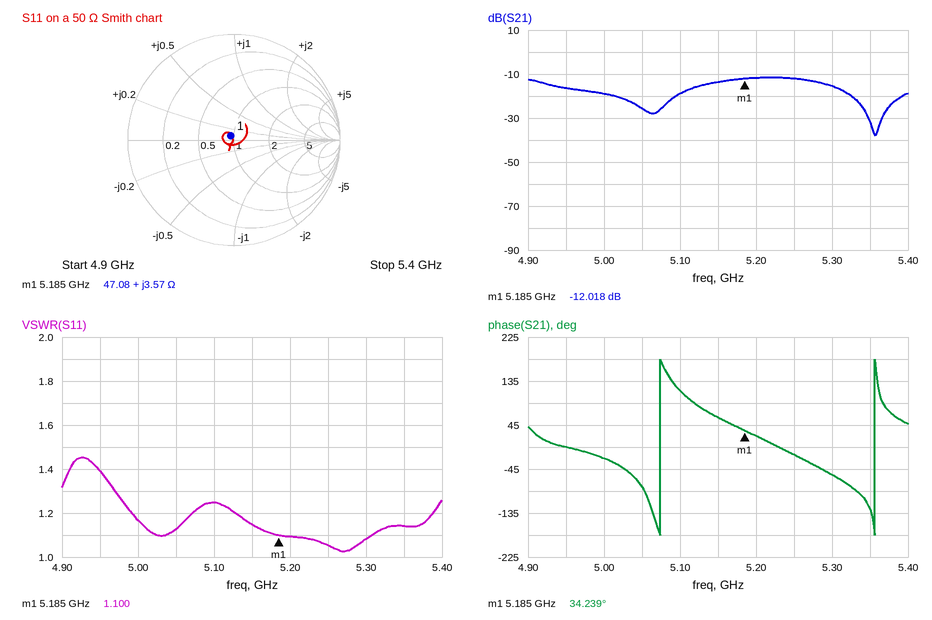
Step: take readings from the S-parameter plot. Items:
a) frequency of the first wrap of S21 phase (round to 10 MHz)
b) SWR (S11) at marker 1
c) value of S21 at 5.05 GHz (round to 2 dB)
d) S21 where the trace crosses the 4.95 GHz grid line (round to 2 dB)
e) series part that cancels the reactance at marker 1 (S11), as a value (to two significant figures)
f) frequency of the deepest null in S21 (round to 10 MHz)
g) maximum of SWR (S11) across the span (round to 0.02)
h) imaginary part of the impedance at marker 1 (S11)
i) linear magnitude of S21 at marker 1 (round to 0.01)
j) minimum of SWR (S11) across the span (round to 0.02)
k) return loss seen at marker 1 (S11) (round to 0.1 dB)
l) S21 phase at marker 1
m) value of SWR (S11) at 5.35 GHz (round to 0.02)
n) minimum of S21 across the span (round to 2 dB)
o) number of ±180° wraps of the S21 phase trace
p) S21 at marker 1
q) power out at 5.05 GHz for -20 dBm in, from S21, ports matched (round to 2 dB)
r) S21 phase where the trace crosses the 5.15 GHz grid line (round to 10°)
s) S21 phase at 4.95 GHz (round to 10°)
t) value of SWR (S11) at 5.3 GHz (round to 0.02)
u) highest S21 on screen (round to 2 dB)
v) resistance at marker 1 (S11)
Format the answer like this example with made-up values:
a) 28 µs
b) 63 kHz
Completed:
a) 5.07 GHz
b) 1.100
c) -26 dB
d) -16 dB
e) 8.6 pF
f) 5.36 GHz
g) 1.46
h) +3.57 Ω
i) 0.25
j) 1.02
k) 26.5 dB
l) 34.239°
m) 1.14
n) -38 dB
o) 2
p) -12.018 dB
q) -46 dBm
r) 60°
s) 0°
t) 1.08
u) -12 dB
v) 47.08 Ω
